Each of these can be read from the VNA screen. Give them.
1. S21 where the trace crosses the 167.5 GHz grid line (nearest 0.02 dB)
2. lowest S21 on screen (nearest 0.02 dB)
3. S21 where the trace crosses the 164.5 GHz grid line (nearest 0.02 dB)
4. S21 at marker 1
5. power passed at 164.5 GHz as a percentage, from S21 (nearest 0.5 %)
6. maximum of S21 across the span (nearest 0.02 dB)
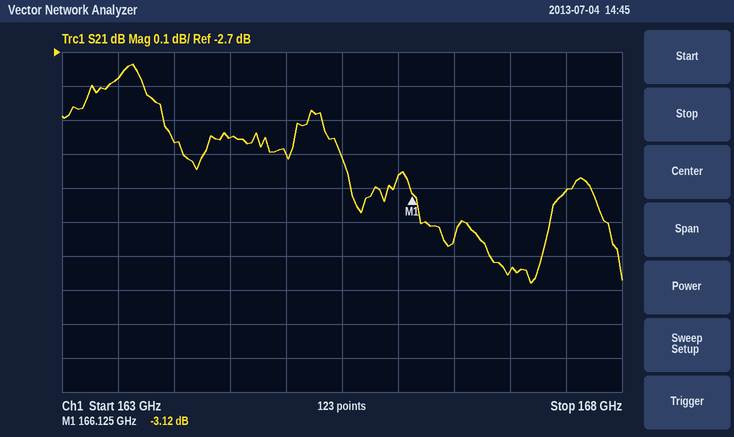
-3.10 dB
-3.38 dB
-2.96 dB
-3.12 dB
50.5 %
-2.74 dB
